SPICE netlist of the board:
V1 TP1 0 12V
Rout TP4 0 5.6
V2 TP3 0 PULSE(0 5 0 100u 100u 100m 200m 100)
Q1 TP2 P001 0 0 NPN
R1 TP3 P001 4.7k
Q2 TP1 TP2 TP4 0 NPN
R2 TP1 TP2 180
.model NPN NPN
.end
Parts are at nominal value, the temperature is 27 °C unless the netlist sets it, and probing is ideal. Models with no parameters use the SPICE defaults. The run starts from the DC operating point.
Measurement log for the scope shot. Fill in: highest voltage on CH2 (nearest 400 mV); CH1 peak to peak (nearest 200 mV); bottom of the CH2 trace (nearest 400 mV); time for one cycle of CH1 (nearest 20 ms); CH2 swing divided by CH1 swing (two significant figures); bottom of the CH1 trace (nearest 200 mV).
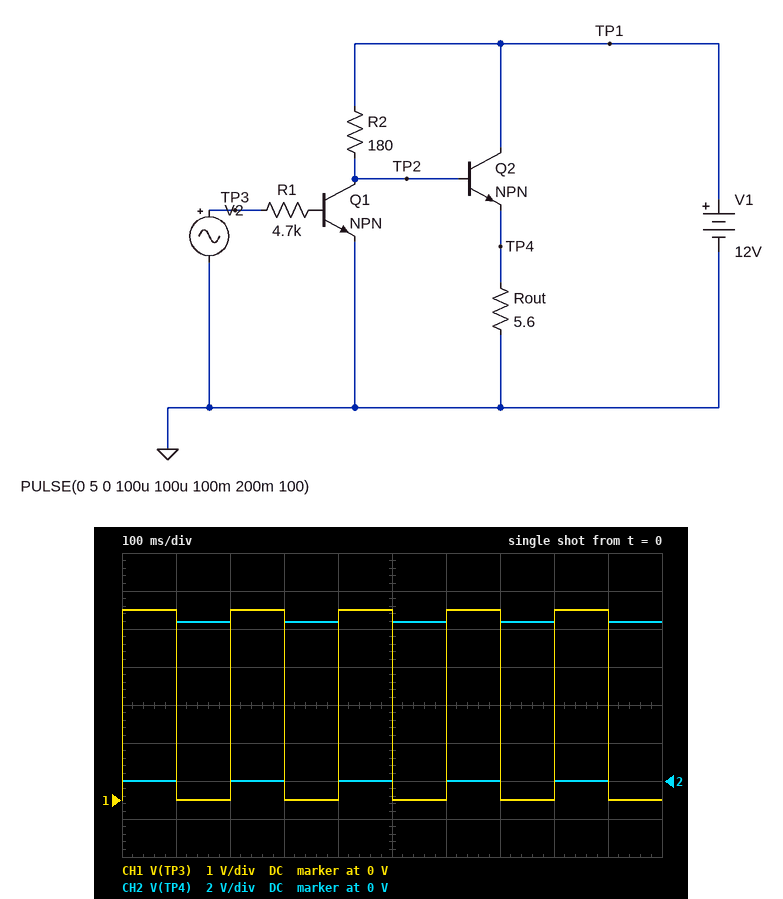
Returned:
8.4 V
5.0 V
0 V
200 ms
1.7
0 V
